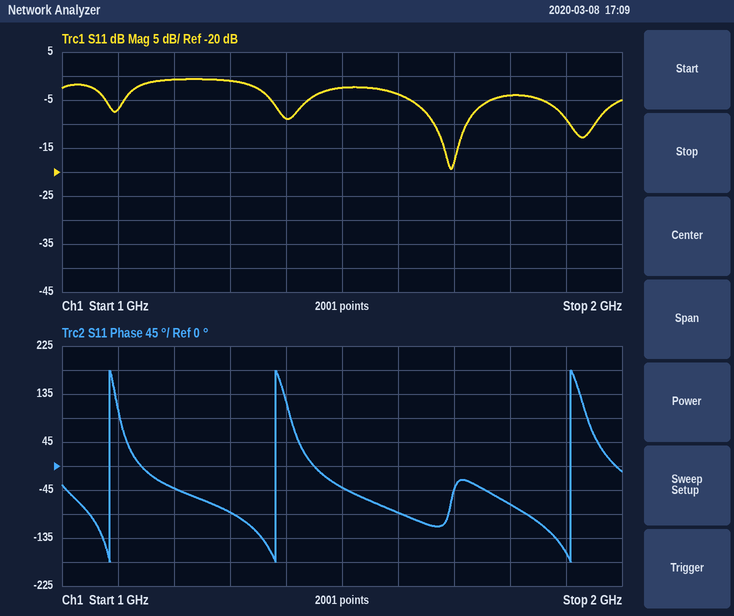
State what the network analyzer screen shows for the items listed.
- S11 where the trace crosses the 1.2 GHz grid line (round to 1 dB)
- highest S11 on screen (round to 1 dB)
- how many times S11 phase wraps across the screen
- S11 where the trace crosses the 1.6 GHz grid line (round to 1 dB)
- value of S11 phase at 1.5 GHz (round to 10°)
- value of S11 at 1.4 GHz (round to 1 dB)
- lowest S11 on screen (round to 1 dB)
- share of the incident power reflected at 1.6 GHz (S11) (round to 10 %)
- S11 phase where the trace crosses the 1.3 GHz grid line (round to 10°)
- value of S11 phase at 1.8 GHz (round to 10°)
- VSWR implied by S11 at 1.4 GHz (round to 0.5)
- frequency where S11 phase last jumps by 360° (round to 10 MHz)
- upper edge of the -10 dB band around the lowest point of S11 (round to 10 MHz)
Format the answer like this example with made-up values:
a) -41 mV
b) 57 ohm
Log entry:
a) -1 dB
b) -1 dB
c) 3
d) -4 dB
e) -40°
f) -9 dB
g) -19 dB
h) 40 %
i) -90°
j) -70°
k) 2.0
l) 1.91 GHz
m) 1.72 GHz
